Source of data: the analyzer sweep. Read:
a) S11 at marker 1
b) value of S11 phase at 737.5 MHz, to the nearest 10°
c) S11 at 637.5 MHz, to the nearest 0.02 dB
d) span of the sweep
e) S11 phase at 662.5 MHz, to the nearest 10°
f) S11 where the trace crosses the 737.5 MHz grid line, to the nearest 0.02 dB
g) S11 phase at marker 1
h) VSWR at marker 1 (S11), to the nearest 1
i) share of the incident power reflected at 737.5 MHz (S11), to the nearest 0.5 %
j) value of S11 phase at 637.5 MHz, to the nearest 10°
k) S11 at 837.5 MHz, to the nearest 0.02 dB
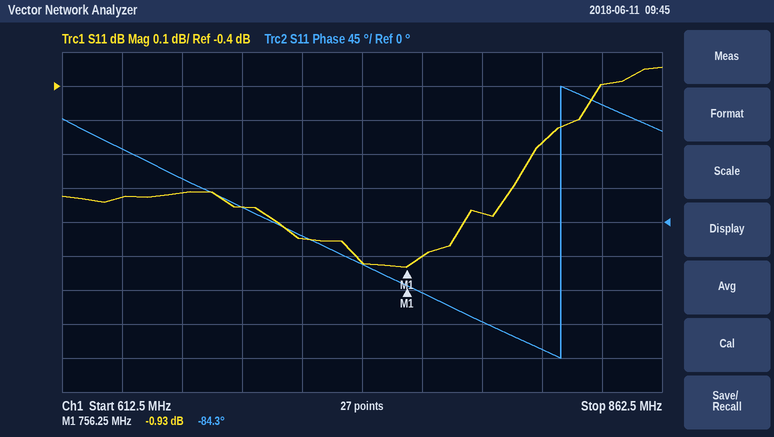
-0.93 dB
-60°
-0.72 dB
250 MHz
60°
-0.92 dB
-84.3°
19
81.0 %
100°
-0.40 dB
